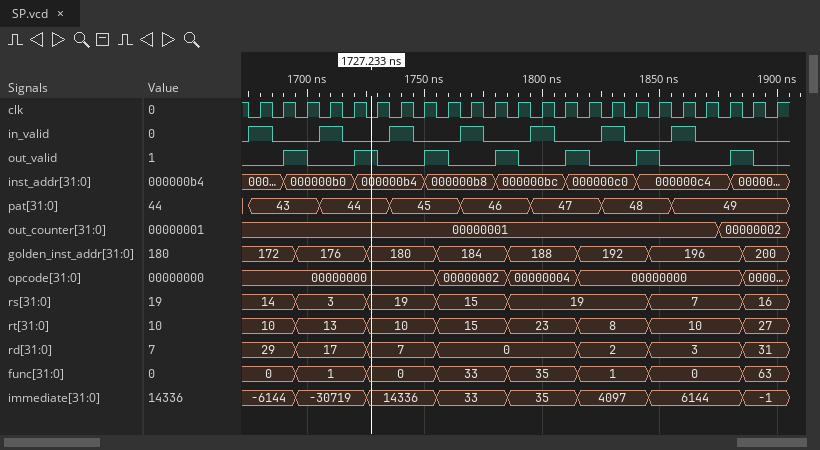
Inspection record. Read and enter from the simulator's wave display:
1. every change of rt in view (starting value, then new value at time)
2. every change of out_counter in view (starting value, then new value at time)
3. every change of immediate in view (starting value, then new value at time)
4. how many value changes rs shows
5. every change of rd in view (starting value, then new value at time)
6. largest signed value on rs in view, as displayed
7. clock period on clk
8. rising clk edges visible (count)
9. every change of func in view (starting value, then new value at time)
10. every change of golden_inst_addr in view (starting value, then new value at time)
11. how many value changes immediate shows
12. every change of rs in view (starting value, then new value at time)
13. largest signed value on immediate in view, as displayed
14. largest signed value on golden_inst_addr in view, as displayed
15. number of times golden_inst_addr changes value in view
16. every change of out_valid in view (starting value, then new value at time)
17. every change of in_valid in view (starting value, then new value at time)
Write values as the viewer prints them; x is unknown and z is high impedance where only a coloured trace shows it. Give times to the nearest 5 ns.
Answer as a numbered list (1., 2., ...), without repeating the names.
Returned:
1. 10, 13 at 1695 ns, 10 at 1725 ns, 15 at 1755 ns, 23 at 1785 ns, 8 at 1815 ns, 10 at 1845 ns, 27 at 1885 ns
2. 00000001, 00000002 at 1875 ns
3. -6144, -30719 at 1695 ns, 14336 at 1725 ns, 33 at 1755 ns, 35 at 1785 ns, 4097 at 1815 ns, 6144 at 1845 ns, -1 at 1885 ns
4. 6
5. 29, 17 at 1695 ns, 7 at 1725 ns, 0 at 1755 ns, 2 at 1815 ns, 3 at 1845 ns, 31 at 1885 ns
6. 19
7. 10 ns
8. 23
9. 0, 1 at 1695 ns, 0 at 1725 ns, 33 at 1755 ns, 35 at 1785 ns, 1 at 1815 ns, 0 at 1845 ns, 63 at 1885 ns
10. 172, 176 at 1695 ns, 180 at 1725 ns, 184 at 1755 ns, 188 at 1785 ns, 192 at 1815 ns, 196 at 1845 ns, 200 at 1885 ns
11. 7
12. 14, 3 at 1695 ns, 19 at 1725 ns, 15 at 1755 ns, 19 at 1785 ns, 7 at 1845 ns, 16 at 1885 ns
13. 14336
14. 200
15. 7
16. 0, 1 at 1690 ns, 0 at 1700 ns, 1 at 1720 ns, 0 at 1730 ns, 1 at 1750 ns, 0 at 1760 ns, 1 at 1780 ns, 0 at 1790 ns, 1 at 1810 ns, 0 at 1820 ns, 1 at 1840 ns, 0 at 1850 ns, 1 at 1880 ns, 0 at 1890 ns
17. 0, 1 at 1675 ns, 0 at 1685 ns, 1 at 1705 ns, 0 at 1715 ns, 1 at 1735 ns, 0 at 1745 ns, 1 at 1765 ns, 0 at 1775 ns, 1 at 1795 ns, 0 at 1805 ns, 1 at 1825 ns, 0 at 1835 ns, 1 at 1855 ns, 0 at 1865 ns
